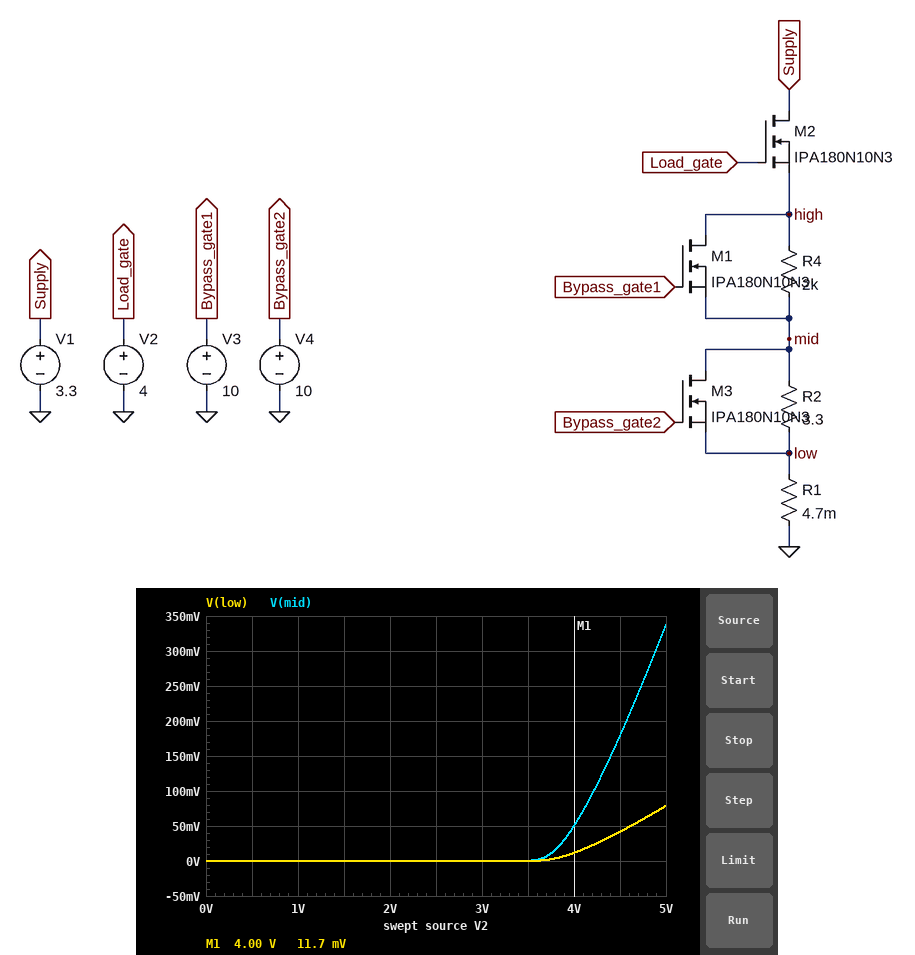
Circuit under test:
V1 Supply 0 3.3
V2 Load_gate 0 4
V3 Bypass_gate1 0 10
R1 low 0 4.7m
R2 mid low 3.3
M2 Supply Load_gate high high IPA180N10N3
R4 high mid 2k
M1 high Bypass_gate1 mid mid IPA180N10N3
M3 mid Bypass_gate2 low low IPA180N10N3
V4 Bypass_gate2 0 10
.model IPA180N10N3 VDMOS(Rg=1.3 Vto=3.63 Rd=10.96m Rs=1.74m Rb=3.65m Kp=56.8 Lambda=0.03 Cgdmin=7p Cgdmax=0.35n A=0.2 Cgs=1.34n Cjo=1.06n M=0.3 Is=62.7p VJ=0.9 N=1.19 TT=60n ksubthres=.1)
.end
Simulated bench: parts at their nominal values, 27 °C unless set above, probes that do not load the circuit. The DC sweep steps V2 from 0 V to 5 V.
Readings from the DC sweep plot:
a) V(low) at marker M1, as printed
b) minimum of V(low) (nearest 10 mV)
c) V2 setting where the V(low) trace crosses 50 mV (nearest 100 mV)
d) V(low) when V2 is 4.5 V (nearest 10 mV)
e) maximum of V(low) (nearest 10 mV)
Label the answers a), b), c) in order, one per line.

a) 11.7 mV
b) 0 V
c) 4.6 V
d) 40 mV
e) 80 mV
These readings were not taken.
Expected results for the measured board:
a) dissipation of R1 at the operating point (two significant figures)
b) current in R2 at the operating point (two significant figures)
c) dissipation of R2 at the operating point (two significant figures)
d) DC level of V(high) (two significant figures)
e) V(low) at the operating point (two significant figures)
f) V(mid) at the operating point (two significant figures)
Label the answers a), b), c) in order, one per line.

a) 29 mW
b) 12 mA
c) 450 µW
d) 89 mV
e) 12 mV
f) 50 mV
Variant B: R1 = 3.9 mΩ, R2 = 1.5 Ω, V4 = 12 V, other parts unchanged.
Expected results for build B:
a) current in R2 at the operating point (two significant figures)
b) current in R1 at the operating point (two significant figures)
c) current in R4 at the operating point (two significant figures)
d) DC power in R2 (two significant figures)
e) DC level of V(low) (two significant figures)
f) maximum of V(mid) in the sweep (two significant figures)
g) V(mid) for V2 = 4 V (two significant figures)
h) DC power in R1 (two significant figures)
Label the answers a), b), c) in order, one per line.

a) 25 mA
b) 2.5 A
c) 20 µA
d) 920 µW
e) 9.9 mV
f) 320 mV
g) 47 mV
h) 25 mW
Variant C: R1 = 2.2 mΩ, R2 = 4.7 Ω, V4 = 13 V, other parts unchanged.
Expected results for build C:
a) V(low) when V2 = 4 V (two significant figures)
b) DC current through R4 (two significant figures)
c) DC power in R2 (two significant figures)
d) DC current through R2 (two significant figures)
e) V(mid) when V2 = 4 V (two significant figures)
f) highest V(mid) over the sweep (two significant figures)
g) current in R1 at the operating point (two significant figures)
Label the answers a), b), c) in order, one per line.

a) 5.7 mV
b) 20 µA
c) 300 µW
d) 8.0 mA
e) 43 mV
f) 300 mV
g) 2.6 A
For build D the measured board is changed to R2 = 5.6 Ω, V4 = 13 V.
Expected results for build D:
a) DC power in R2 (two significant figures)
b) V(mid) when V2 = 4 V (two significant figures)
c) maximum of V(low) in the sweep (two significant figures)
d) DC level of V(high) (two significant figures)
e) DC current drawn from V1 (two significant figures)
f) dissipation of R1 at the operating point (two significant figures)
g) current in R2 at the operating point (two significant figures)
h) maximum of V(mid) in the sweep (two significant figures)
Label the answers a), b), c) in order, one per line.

a) 240 µW
b) 48 mV
c) 80 mV
d) 87 mV
e) 2.5 A
f) 30 mW
g) 6.5 mA
h) 330 mV
